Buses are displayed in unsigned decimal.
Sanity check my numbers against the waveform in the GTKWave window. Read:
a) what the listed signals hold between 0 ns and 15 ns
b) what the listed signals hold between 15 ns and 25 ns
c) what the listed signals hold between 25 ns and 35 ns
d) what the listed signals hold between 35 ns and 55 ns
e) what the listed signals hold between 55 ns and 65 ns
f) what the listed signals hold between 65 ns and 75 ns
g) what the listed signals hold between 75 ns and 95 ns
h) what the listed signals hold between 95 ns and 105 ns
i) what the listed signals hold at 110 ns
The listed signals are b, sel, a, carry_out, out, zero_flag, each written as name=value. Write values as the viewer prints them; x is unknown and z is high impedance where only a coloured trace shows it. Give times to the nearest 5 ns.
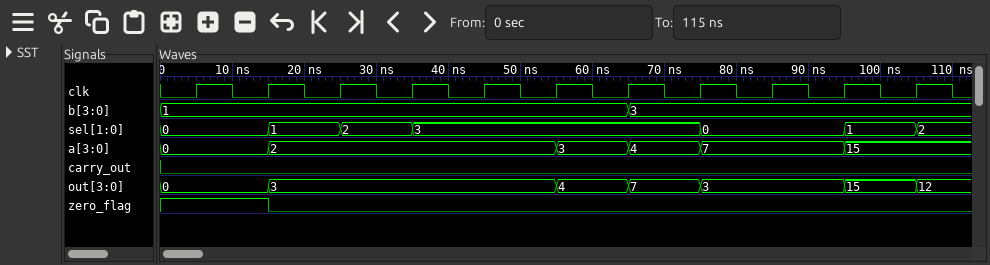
b=1, sel=0, a=0, carry_out=0, out=0, zero_flag=1
b=1, sel=1, a=2, carry_out=0, out=3, zero_flag=0
b=1, sel=2, a=2, carry_out=0, out=3, zero_flag=0
b=1, sel=3, a=2, carry_out=0, out=3, zero_flag=0
b=1, sel=3, a=3, carry_out=0, out=4, zero_flag=0
b=3, sel=3, a=4, carry_out=0, out=7, zero_flag=0
b=3, sel=0, a=7, carry_out=0, out=3, zero_flag=0
b=3, sel=1, a=15, carry_out=0, out=15, zero_flag=0
b=3, sel=2, a=15, carry_out=0, out=12, zero_flag=0
